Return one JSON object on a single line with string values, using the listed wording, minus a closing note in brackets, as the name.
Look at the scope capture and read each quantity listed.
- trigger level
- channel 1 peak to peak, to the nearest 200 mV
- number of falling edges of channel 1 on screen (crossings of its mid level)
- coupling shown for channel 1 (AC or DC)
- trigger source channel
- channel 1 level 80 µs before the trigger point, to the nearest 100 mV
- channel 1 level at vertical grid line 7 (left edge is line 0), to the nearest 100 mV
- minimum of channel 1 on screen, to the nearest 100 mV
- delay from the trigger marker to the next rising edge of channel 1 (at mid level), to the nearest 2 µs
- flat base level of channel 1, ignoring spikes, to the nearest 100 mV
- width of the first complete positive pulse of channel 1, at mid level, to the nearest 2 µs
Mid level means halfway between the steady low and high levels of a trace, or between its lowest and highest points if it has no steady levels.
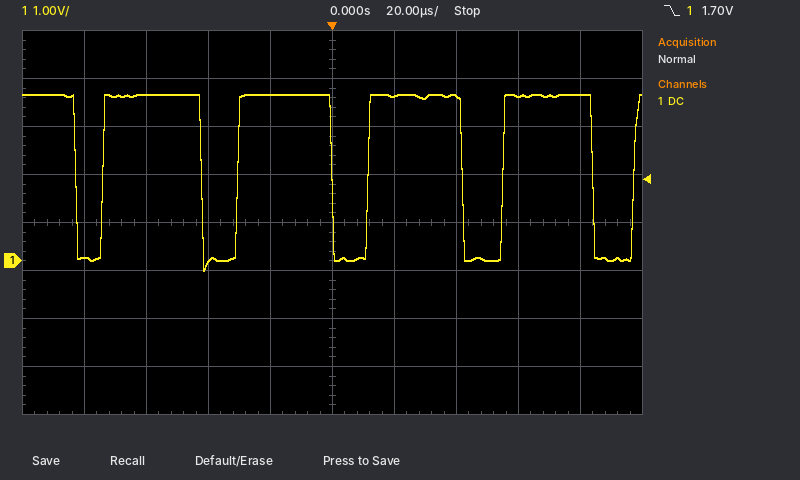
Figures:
{"trigger level": "1.70 V", "channel 1 peak to peak, to the nearest 200 mV": "3.6 V", "number of falling edges of channel 1 on screen": "5", "coupling shown for channel 1": "DC", "trigger source channel": "channel 1", "channel 1 level 80 µs before the trigger point, to the nearest 100 mV": "100 mV", "channel 1 level at vertical grid line 7 (left edge is line 0), to the nearest 100 mV": "3.4 V", "minimum of channel 1 on screen, to the nearest 100 mV": "-200 mV", "delay from the trigger marker to the next rising edge of channel 1 (at mid level), to the nearest 2 µs": "12 µs", "flat base level of channel 1, ignoring spikes, to the nearest 100 mV": "0.0 V", "width of the first complete positive pulse of channel 1, at mid level, to the nearest 2 µs": "32 µs"}
